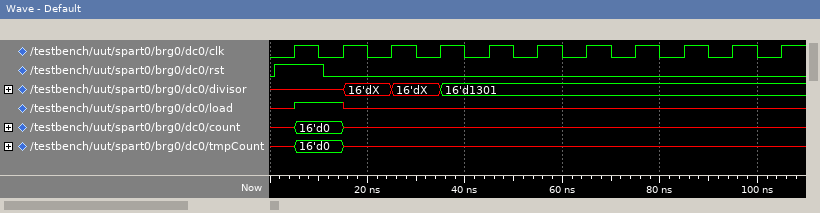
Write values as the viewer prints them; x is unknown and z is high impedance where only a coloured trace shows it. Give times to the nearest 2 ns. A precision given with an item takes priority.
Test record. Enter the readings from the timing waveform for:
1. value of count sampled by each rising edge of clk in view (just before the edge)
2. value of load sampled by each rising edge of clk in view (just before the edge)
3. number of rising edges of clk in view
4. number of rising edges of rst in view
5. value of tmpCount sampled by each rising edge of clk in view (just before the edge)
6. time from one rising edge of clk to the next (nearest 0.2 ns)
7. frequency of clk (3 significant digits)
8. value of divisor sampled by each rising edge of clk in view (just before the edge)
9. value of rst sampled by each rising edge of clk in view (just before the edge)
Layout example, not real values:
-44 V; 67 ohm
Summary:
x, 16'd0, x, x, x, x, x, x, x, x, x; x 1 x x x x x x x x x; 11; 1; x, 16'd0, x, x, x, x, x, x, x, x, x; 10 ns; 100 MHz; x, x, 16'dX, 16'dX, 16'd1301, 16'd1301, 16'd1301, 16'd1301, 16'd1301, 16'd1301, 16'd1301; 1 0 0 0 0 0 0 0 0 0 0
